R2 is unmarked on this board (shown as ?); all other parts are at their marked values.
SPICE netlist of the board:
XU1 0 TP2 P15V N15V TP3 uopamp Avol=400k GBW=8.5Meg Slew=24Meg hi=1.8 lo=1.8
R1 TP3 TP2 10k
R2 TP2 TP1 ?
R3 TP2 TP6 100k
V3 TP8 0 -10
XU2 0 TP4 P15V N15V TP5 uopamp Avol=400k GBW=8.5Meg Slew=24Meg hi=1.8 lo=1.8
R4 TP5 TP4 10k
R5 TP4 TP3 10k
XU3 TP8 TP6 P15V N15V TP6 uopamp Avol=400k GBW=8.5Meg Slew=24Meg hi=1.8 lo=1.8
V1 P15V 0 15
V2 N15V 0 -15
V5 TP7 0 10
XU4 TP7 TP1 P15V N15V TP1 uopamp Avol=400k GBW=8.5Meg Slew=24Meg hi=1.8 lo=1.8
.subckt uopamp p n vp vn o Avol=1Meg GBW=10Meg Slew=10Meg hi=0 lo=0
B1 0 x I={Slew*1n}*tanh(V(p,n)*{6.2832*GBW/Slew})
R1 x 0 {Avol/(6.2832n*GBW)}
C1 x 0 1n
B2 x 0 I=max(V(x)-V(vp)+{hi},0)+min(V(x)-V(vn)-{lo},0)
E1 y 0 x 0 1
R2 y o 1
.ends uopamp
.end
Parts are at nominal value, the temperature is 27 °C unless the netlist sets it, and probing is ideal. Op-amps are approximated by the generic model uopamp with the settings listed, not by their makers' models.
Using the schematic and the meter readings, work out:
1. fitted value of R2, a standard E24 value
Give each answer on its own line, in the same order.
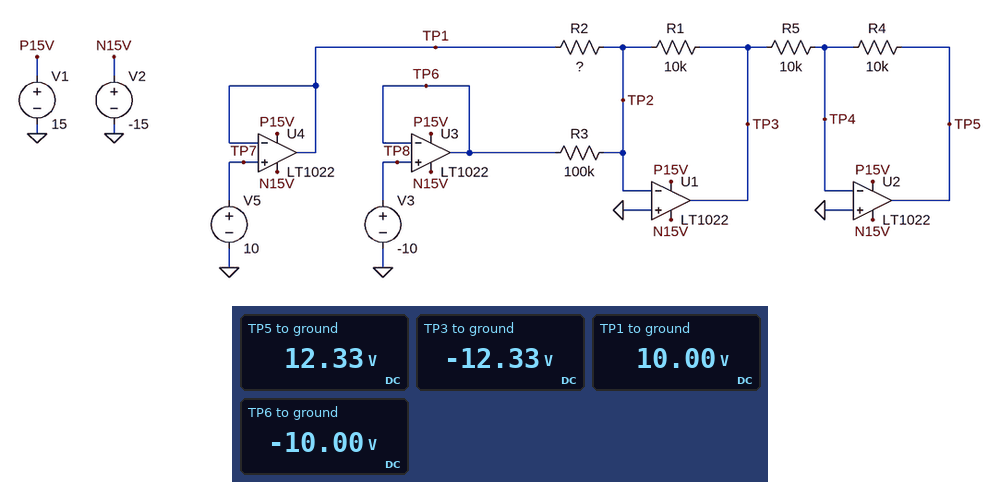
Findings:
7.5 kΩ
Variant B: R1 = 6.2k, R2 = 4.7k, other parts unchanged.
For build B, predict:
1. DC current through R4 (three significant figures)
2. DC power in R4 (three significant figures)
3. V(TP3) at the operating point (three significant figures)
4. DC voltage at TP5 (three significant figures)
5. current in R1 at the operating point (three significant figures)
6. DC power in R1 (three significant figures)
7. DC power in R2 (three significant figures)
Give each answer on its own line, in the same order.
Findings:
1.26 mA
15.8 mW
-12.6 V
12.6 V
2.03 mA
25.5 mW
21.3 mW
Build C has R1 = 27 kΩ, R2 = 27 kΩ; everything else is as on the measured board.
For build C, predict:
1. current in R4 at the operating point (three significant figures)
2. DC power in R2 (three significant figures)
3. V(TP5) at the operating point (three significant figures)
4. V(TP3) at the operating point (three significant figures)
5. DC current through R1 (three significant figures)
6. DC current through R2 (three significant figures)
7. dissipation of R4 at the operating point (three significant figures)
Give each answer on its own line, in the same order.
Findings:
730 µA
3.70 mW
7.30 V
-7.30 V
270 µA
370 µA
5.33 mW
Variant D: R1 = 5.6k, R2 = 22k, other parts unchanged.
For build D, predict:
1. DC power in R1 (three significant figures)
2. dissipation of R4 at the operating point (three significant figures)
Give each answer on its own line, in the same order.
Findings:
704 µW
394 µW
